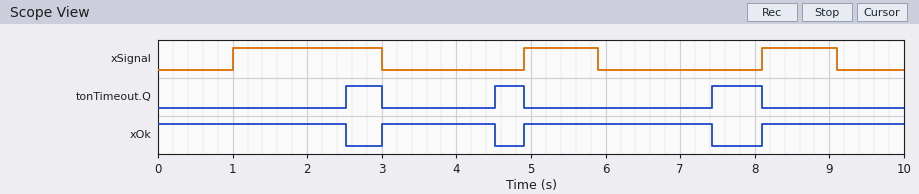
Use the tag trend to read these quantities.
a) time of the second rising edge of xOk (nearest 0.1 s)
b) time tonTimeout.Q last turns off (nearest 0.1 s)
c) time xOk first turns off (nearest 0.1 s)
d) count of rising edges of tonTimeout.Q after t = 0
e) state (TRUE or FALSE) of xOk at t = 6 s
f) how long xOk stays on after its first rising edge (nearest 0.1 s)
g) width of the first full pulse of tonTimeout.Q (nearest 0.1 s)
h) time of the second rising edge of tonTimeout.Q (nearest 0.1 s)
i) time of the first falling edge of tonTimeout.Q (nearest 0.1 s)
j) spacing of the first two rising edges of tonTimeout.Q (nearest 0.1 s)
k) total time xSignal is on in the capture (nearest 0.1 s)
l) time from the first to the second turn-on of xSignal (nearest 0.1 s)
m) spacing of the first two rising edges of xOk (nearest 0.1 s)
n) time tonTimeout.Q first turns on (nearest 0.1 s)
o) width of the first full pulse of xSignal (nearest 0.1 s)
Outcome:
4.9 s
8.1 s
2.5 s
3
TRUE
1.5 s
0.5 s
4.5 s
3.0 s
2.0 s
4.0 s
3.9 s
1.9 s
2.5 s
2.0 s
